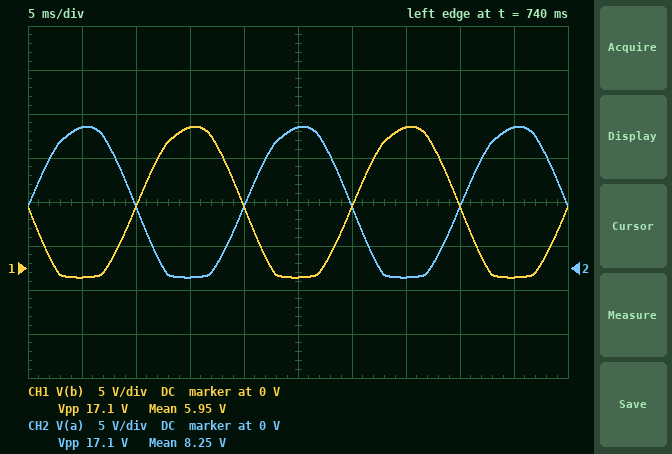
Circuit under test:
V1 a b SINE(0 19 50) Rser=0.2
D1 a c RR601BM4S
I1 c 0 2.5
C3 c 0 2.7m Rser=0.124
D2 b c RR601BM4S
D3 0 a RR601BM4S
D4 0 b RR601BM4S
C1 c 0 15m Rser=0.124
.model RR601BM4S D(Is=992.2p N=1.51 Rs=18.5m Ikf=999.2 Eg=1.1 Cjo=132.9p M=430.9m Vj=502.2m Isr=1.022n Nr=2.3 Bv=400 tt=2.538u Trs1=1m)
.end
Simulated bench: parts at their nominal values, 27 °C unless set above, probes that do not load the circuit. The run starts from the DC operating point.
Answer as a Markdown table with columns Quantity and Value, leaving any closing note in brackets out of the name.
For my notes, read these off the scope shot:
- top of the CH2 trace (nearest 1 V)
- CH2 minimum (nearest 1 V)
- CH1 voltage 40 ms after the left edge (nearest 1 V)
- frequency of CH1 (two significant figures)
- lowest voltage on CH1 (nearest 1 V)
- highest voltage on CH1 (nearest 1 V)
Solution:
| Quantity | Value |
|---|---|
| top of the CH2 trace | 16 V |
| CH2 minimum | -1 V |
| CH1 voltage 40 ms after the left edge | 7 V |
| frequency of CH1 | 50 Hz |
| lowest voltage on CH1 | -1 V |
| highest voltage on CH1 | 16 V |
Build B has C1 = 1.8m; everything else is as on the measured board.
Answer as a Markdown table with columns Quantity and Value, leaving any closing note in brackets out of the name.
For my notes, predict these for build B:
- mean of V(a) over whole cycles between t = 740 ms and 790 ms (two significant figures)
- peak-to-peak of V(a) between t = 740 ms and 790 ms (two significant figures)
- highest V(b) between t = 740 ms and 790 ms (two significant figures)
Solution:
| Quantity | Value |
|---|---|
| mean of V(a) over whole cycles between t = 740 ms and 790 ms | 7.0 V |
| peak-to-peak of V(a) between t = 740 ms and 790 ms | 18 V |
| highest V(b) between t = 740 ms and 790 ms | 17 V |
